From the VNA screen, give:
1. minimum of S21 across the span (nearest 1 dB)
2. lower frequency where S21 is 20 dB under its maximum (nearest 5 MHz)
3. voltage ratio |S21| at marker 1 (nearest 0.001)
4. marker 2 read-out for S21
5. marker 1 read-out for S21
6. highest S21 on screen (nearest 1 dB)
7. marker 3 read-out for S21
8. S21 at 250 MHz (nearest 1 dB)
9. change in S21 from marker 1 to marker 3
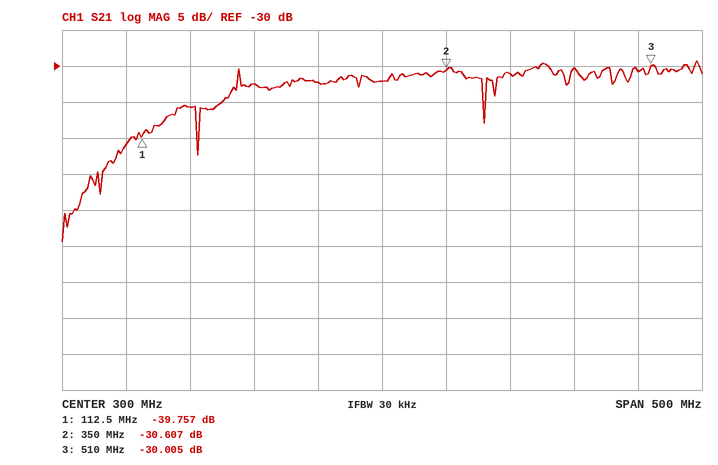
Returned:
-54 dB
65 MHz
0.010
-30.607 dB
-39.757 dB
-29 dB
-30.005 dB
-32 dB
9.752 dB
